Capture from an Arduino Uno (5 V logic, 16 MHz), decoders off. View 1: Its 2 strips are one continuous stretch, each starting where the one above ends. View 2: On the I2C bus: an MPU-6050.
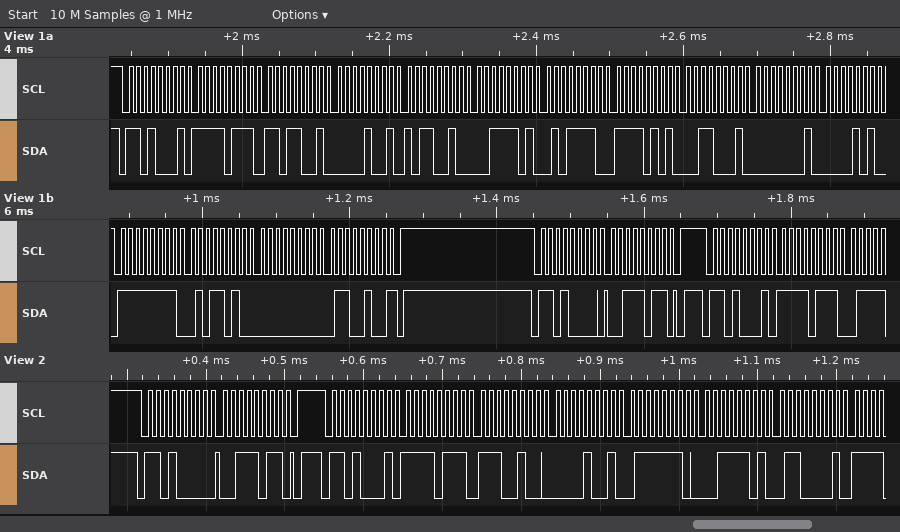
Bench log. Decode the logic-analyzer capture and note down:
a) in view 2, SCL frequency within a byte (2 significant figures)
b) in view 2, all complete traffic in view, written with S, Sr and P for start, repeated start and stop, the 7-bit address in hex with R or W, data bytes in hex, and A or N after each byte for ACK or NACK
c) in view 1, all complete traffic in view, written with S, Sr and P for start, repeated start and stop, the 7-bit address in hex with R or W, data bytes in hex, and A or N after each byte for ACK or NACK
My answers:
100 kHz
S 68W A 3B A P S 68R A F7 A E4 A 09 A 7E A 3D A 61 A
S 68R A F7 A D9 A 09 A B2 A 3D A 5E A F5 A 31 A 01 A 0A A FF A 5A A 00 A 64 N P S 68W A 3B A P S 68R A F7 A
